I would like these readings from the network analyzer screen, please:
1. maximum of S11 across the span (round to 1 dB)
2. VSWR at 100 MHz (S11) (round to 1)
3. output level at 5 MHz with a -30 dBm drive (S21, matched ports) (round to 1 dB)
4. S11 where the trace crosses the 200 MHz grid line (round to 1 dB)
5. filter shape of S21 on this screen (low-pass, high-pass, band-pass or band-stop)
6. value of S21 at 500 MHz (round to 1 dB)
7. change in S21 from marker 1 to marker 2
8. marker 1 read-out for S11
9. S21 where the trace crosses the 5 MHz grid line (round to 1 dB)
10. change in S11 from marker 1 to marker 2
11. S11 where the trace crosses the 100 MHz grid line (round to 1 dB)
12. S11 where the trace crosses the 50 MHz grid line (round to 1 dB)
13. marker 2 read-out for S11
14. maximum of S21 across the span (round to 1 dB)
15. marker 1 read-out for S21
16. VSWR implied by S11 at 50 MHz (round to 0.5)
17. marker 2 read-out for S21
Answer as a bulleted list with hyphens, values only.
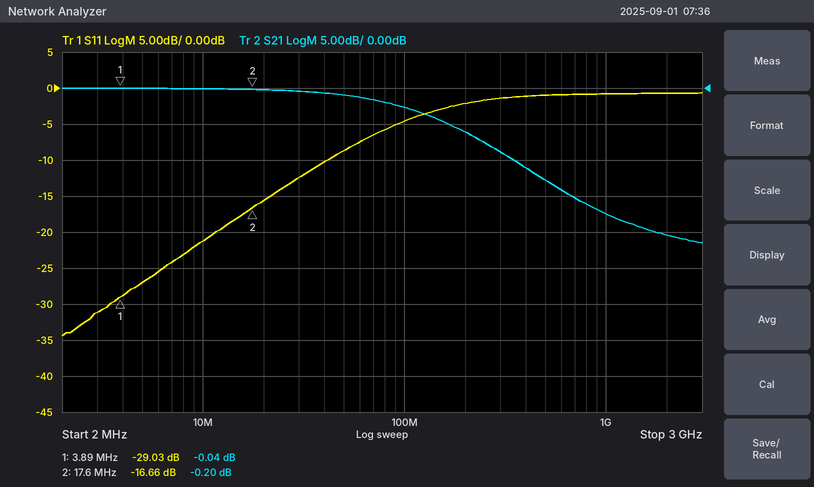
- -1 dB
- 4
- -30 dBm
- -2 dB
- low-pass
- -13 dB
- -0.16 dB
- -29.03 dB
- 0 dB
- 12.37 dB
- -5 dB
- -9 dB
- -16.66 dB
- 0 dB
- -0.04 dB
- 2.0
- -0.20 dB
